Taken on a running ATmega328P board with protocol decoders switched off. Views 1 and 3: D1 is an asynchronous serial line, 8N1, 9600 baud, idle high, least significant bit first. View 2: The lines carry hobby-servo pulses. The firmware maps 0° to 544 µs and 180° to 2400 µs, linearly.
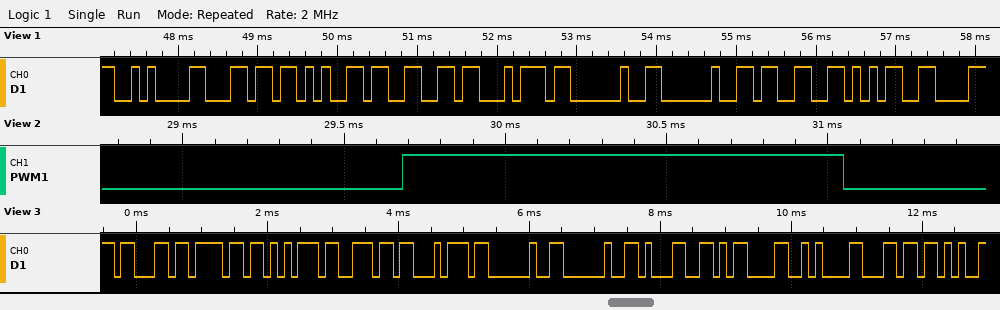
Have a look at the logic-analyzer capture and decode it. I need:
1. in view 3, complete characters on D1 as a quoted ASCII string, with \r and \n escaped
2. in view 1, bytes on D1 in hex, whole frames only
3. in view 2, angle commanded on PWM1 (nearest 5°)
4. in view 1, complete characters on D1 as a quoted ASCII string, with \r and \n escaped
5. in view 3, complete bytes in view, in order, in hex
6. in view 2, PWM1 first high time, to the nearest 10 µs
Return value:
"count  1\r\nl"
0A 6C 65 66 74 20 20 33 35
80°
"\nleft  35"
0x63 0x6F 0x75 0x6E 0x74 0x20 0x20 0x31 0x0D 0x0A 0x6C
1370 µs
